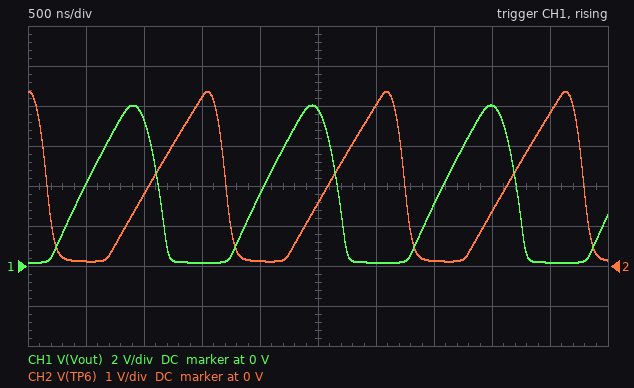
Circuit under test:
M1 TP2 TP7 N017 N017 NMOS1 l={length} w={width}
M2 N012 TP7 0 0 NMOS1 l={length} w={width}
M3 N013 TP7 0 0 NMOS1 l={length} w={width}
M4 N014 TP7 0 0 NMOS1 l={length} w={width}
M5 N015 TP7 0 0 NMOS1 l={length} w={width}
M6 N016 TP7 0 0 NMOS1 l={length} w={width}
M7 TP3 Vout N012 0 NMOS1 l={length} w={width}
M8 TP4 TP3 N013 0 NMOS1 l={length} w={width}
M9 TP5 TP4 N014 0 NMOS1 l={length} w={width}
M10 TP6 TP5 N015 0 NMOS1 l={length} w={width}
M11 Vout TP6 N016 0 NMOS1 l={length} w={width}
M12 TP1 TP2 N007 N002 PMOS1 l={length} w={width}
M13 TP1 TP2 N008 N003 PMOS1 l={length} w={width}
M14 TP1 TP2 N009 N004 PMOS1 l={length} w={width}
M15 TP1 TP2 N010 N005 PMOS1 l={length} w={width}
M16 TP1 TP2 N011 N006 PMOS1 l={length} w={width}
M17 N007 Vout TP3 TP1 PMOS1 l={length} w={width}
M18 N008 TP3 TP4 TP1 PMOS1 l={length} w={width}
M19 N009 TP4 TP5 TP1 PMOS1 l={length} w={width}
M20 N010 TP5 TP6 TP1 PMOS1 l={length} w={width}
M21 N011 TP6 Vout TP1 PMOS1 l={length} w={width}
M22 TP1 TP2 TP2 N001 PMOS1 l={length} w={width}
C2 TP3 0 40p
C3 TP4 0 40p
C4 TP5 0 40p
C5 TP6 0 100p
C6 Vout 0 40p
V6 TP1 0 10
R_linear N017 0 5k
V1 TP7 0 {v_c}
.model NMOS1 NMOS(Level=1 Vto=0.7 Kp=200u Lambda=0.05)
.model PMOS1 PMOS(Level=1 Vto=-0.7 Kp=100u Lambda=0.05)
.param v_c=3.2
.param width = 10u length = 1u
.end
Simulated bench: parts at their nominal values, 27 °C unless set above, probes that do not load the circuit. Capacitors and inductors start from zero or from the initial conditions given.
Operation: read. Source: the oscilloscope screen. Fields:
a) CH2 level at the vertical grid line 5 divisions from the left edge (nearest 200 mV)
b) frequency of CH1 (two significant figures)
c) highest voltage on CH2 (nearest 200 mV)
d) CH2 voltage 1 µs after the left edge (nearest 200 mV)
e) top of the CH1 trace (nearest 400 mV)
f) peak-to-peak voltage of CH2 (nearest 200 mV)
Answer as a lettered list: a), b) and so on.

a) 1.6 V
b) 650 kHz
c) 4.4 V
d) 1.8 V
e) 8.0 V
f) 4.2 V
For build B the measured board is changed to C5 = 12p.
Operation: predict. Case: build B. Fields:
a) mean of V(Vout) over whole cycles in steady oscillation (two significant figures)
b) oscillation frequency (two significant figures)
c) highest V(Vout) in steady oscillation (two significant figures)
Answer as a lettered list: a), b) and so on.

a) 2.0 V
b) 1.0 MHz
c) 6.1 V
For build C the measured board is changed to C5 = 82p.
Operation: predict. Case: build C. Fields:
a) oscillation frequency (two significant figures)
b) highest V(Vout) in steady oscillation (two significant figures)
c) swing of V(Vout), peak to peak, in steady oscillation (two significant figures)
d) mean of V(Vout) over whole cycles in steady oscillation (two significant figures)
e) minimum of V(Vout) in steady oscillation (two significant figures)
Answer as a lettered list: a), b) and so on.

a) 690 kHz
b) 7.7 V
c) 7.5 V
d) 3.0 V
e) 140 mV
